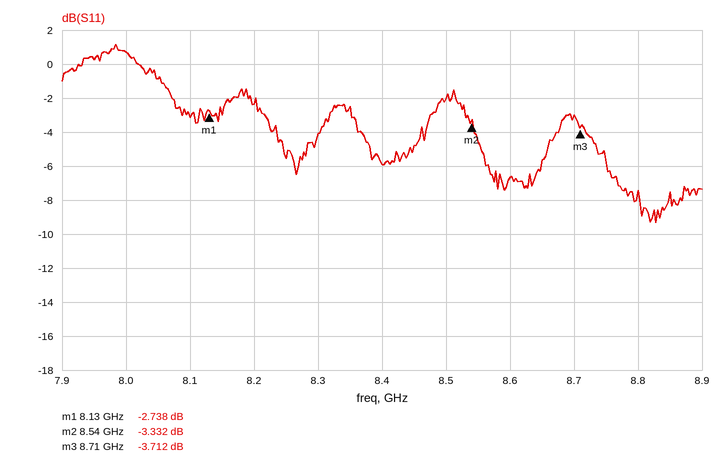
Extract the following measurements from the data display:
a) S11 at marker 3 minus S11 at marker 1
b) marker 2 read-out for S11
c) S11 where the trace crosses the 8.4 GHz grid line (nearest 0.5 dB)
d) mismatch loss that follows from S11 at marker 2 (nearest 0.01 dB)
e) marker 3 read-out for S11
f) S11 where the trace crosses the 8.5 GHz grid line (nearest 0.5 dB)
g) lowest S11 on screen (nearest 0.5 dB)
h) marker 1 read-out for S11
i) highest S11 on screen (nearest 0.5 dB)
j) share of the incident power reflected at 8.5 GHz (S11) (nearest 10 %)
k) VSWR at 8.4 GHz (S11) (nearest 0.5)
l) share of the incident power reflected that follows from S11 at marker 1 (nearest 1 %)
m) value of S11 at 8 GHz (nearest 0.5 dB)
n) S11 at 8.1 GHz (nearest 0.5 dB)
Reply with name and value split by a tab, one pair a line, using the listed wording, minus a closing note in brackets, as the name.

S11 at marker 3 minus S11 at marker 1	-0.974 dB
marker 2 read-out for S11	-3.332 dB
S11 where the trace crosses the 8.4 GHz grid line	-6.0 dB
mismatch loss that follows from S11 at marker 2	2.71 dB
marker 3 read-out for S11	-3.712 dB
S11 where the trace crosses the 8.5 GHz grid line	-2.0 dB
lowest S11 on screen	-9.5 dB
marker 1 read-out for S11	-2.738 dB
highest S11 on screen	1.0 dB
share of the incident power reflected at 8.5 GHz (S11)	60 %
VSWR at 8.4 GHz (S11)	3.0
share of the incident power reflected that follows from S11 at marker 1	53 %
value of S11 at 8 GHz	0.5 dB
S11 at 8.1 GHz	-3.0 dB
